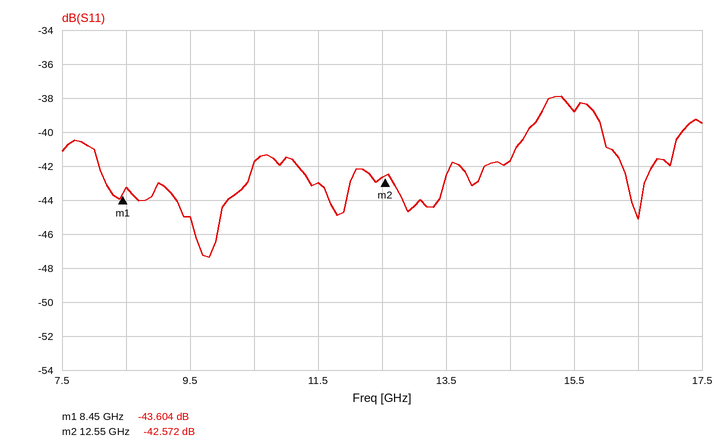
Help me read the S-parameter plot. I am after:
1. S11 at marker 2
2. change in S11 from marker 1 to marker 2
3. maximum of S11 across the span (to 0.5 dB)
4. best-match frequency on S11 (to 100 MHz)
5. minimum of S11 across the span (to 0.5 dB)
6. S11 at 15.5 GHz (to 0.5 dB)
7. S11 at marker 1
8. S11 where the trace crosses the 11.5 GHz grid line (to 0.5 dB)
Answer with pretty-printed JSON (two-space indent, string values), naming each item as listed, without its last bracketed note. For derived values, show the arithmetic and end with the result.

{
  "S11 at marker 2": "-42.572 dB",
  "change in S11 from marker 1 to marker 2": "-42.572 − (-43.604) = 1.032 dB",
  "maximum of S11 across the span": "-38.0 dB",
  "best-match frequency on S11": "9.8 GHz",
  "minimum of S11 across the span": "-47.5 dB",
  "S11 at 15.5 GHz": "-39.0 dB",
  "S11 at marker 1": "-43.604 dB",
  "S11 where the trace crosses the 11.5 GHz grid line": "-43.0 dB"
}
